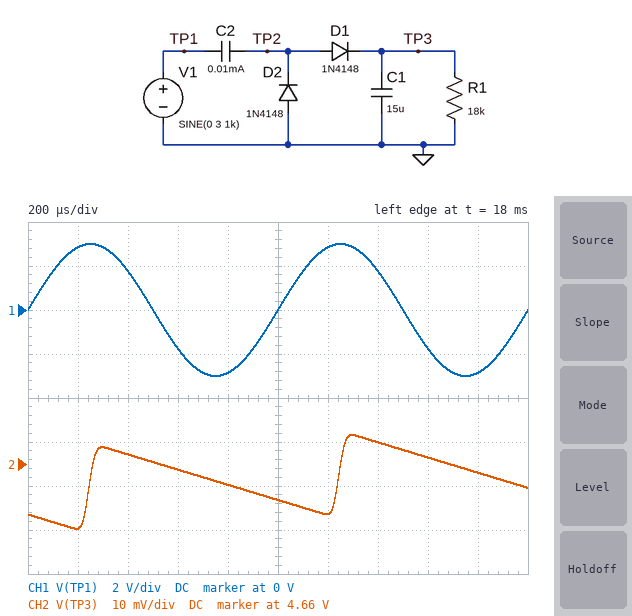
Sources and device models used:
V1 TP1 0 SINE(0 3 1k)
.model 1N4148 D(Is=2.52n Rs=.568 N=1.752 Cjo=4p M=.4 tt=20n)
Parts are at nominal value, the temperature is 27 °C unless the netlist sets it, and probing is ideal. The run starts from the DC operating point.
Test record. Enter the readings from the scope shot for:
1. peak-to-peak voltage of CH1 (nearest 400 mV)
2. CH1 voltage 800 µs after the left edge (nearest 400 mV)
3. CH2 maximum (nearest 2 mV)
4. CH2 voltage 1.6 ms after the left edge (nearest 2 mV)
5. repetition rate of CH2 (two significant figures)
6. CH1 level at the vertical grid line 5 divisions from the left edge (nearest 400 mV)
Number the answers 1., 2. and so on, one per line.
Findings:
1. 6.0 V
2. -2.8 V
3. 4.666 V
4. 4.662 V
5. 1.0 kHz
6. 0 V
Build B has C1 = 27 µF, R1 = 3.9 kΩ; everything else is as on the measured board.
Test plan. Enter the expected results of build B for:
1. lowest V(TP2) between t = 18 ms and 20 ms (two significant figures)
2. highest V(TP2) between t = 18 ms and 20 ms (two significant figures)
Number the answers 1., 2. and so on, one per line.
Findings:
1. -740 mV
2. 5.2 V
